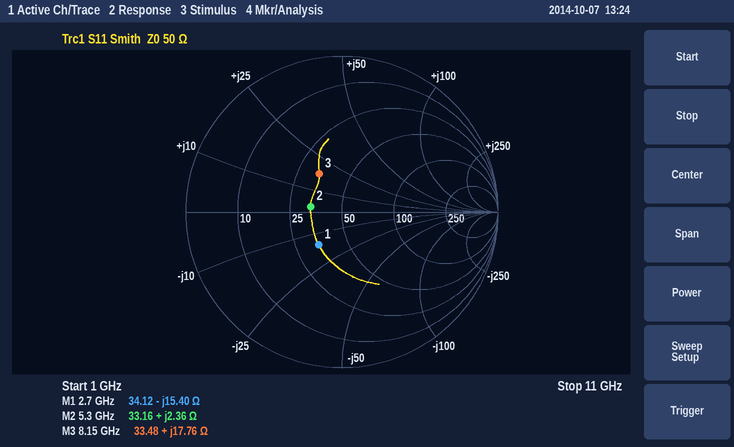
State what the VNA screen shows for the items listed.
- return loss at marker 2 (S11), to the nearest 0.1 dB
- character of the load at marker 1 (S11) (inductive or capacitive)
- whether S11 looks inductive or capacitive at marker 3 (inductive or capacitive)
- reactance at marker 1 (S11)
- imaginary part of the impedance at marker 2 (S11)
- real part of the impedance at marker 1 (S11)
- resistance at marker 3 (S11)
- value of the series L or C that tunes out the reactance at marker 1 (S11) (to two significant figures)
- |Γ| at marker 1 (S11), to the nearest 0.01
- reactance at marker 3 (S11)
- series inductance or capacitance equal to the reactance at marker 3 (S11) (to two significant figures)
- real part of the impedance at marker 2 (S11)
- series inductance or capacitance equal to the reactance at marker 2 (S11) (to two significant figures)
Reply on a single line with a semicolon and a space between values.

13.8 dB; capacitive; inductive; -15.40 Ω; +2.36 Ω; 34.12 Ω; 33.48 Ω; 910 pH; 0.26; +17.76 Ω; 350 pH; 33.16 Ω; 71 pH
